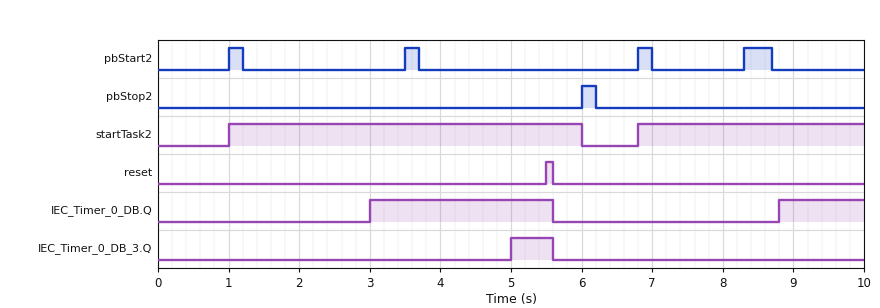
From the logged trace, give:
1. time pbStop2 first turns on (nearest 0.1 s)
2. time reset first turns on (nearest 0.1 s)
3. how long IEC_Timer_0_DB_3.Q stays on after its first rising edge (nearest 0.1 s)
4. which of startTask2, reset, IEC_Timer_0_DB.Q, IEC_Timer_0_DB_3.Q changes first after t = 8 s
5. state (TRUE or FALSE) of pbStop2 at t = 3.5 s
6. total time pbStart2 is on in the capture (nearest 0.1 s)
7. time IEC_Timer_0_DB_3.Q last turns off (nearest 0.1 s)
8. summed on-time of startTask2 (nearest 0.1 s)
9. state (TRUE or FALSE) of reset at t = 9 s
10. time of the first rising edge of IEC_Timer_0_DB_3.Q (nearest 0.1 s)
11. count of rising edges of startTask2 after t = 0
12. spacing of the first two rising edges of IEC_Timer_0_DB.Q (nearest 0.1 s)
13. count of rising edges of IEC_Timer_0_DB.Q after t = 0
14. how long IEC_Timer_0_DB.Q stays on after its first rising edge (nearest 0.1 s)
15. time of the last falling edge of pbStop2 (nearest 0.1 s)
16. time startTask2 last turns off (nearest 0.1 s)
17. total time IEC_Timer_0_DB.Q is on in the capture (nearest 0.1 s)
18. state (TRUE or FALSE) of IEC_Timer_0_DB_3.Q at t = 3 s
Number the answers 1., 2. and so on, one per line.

1. 6.0 s
2. 5.5 s
3. 0.6 s
4. IEC_Timer_0_DB.Q
5. FALSE
6. 1.0 s
7. 5.6 s
8. 8.2 s
9. FALSE
10. 5.0 s
11. 2
12. 5.8 s
13. 2
14. 2.6 s
15. 6.2 s
16. 6.0 s
17. 3.8 s
18. FALSE
